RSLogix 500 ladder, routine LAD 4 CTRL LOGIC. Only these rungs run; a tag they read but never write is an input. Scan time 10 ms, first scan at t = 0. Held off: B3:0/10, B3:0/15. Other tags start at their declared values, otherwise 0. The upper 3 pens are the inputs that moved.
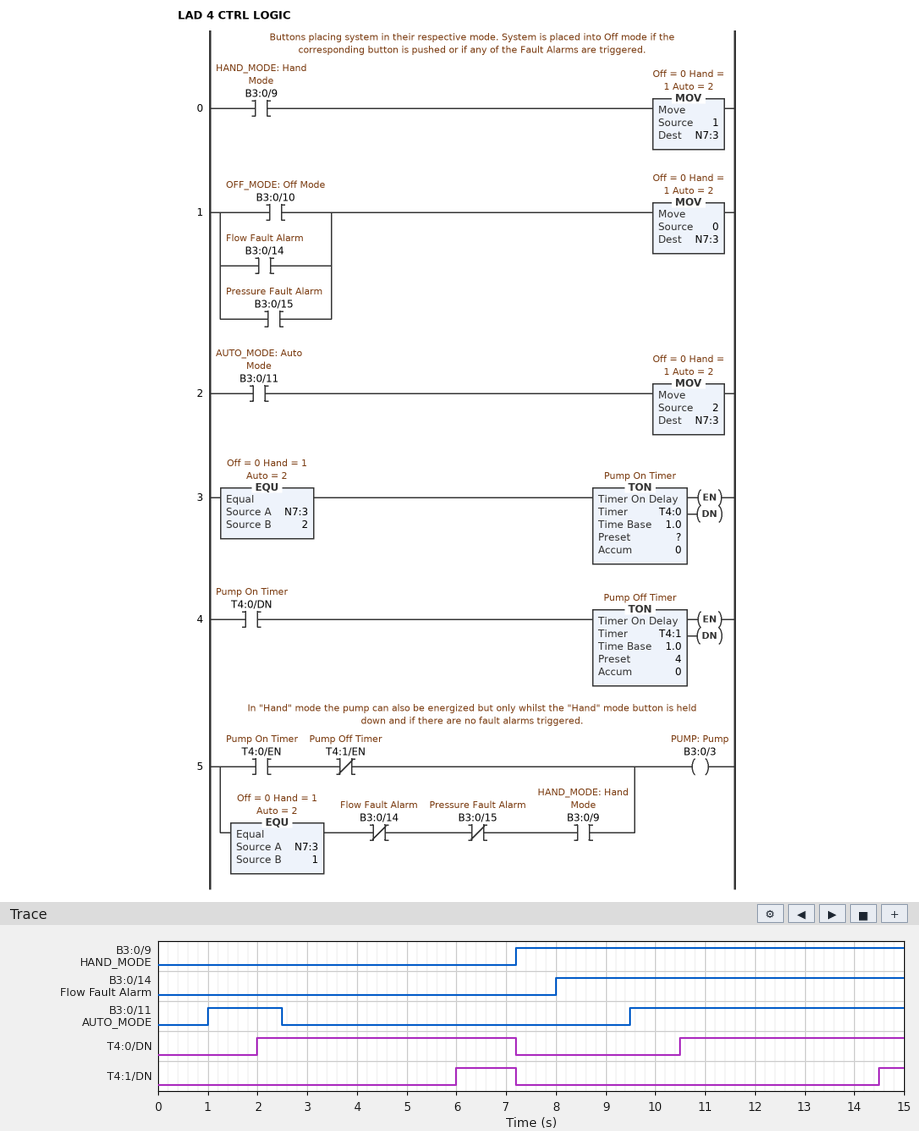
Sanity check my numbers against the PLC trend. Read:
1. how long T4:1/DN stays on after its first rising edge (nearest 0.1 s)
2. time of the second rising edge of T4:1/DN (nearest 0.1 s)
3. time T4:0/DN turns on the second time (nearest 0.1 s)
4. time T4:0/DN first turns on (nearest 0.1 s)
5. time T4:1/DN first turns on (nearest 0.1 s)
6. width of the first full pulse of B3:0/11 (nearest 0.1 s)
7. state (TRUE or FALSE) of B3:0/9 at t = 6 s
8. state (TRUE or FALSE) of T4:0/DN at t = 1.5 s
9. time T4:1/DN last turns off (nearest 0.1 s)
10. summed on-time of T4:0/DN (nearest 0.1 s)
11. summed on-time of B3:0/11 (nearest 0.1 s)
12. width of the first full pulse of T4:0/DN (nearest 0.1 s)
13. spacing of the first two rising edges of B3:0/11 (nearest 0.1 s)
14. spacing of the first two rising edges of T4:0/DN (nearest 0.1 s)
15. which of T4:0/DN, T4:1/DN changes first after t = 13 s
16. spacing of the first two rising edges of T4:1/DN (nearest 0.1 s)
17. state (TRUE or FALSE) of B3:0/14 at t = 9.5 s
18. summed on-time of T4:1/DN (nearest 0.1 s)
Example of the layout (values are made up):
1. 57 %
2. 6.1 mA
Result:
1. 1.2 s
2. 14.5 s
3. 10.5 s
4. 2.0 s
5. 6.0 s
6. 1.5 s
7. FALSE
8. FALSE
9. 7.2 s
10. 9.7 s
11. 7.0 s
12. 5.2 s
13. 8.5 s
14. 8.5 s
15. T4:1/DN
16. 8.5 s
17. TRUE
18. 1.7 s
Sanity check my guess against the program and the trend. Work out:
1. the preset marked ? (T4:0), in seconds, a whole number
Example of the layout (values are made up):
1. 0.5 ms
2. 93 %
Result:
1. 1 s
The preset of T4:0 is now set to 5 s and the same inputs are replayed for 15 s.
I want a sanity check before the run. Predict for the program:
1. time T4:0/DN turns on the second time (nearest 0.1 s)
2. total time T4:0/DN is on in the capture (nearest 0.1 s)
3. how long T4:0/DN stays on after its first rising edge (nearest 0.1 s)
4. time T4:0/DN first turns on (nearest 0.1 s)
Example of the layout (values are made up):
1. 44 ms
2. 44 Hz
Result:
1. 14.5 s
2. 1.7 s
3. 1.2 s
4. 6.0 s
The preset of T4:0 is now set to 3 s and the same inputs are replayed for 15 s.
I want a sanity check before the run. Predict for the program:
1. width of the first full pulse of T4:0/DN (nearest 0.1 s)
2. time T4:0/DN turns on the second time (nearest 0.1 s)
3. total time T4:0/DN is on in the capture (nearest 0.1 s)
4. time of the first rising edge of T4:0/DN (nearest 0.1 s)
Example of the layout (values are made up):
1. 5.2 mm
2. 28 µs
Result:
1. 3.2 s
2. 12.5 s
3. 5.7 s
4. 4.0 s
